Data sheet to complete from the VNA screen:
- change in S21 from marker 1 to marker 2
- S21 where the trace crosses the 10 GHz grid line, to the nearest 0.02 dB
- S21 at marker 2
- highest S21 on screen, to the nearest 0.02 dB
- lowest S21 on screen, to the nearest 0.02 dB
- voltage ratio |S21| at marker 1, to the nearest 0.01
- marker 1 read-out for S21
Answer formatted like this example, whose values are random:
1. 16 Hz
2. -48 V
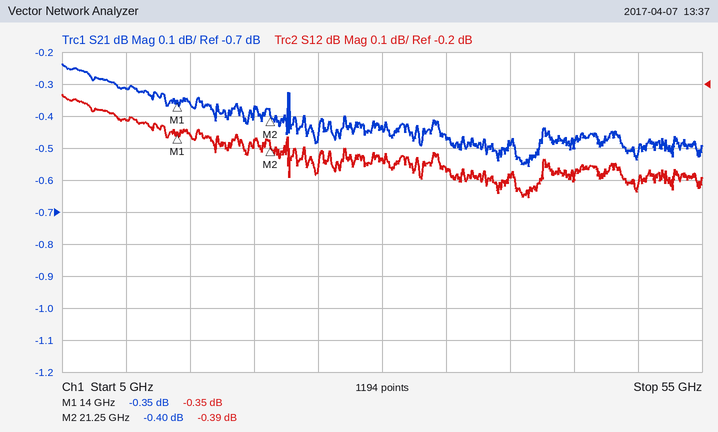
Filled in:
1. -0.05 dB
2. -0.32 dB
3. -0.40 dB
4. -0.24 dB
5. -0.56 dB
6. 0.96
7. -0.35 dB
